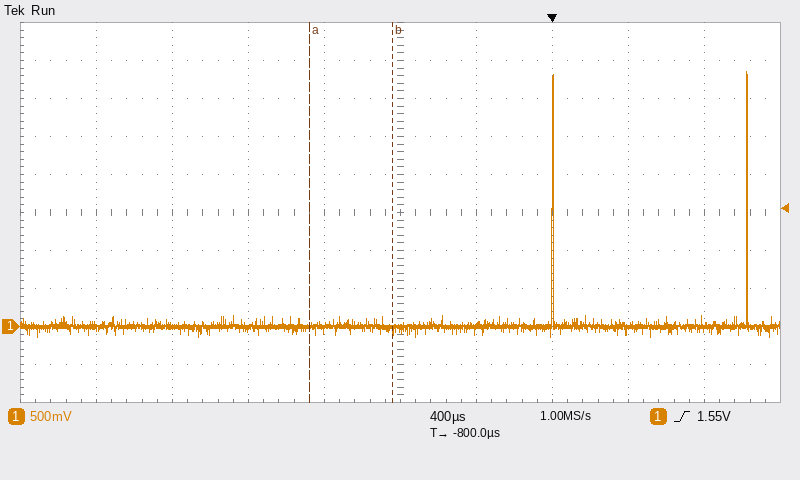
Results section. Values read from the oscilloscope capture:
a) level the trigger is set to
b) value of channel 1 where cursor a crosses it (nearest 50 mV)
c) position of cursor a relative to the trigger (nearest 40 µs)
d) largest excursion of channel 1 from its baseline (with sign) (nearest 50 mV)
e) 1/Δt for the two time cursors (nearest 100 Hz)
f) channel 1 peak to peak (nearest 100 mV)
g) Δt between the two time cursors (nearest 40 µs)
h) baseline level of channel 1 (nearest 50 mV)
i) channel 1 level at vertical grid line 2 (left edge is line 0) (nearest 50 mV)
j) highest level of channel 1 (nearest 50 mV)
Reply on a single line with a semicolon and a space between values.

1.55 V; 0 mV; -1.28 ms; +3.35 V; 2.3 kHz; 3.50 V; 440 µs; 0 mV; 0 mV; 3.35 V
